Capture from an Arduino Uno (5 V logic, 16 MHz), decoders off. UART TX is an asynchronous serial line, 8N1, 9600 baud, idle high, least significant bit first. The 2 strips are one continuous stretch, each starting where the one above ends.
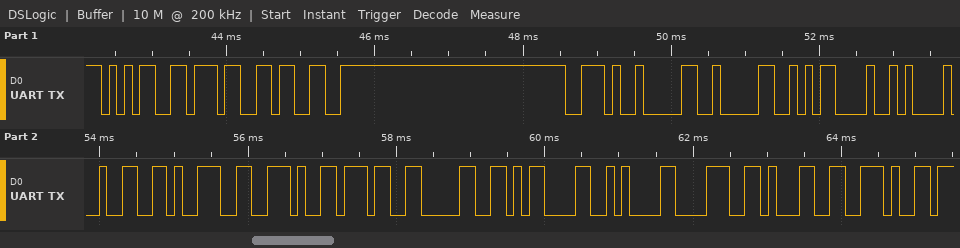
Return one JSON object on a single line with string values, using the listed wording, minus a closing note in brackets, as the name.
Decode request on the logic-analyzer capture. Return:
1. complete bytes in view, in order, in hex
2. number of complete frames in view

{"complete bytes in view, in order, in hex": "35 37 33 2E 30 30 0D 0A 32 39 2E 37 30 0D 0A 38 31 2E", "number of complete frames in view": "18"}
